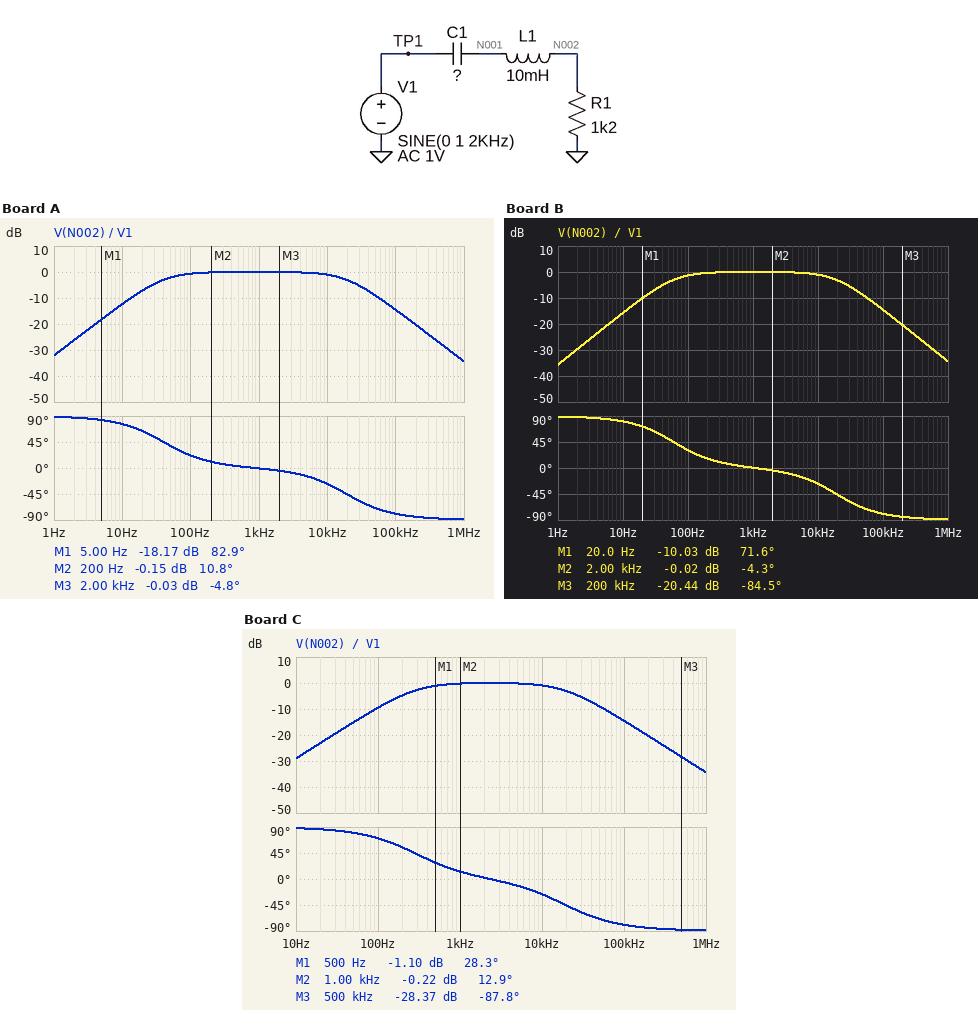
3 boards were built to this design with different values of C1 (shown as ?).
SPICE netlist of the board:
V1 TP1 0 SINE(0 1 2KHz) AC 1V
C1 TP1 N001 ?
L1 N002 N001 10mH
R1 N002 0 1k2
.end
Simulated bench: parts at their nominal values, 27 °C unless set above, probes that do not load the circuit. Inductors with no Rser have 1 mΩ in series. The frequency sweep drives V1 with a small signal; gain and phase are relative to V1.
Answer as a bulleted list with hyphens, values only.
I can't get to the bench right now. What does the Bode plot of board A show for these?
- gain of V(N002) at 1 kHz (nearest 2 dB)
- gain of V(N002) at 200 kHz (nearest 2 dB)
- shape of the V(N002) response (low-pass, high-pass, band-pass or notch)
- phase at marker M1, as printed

- 0 dB
- -20 dB
- band-pass
- 82.9 deg
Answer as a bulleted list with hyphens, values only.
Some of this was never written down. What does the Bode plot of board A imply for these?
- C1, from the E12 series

- 3.3 µF
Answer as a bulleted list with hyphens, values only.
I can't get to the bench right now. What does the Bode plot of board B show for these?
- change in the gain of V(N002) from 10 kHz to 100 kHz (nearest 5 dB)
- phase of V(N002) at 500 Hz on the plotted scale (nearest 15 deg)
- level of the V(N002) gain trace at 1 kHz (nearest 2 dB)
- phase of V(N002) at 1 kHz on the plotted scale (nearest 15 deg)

- -15 dB
- 0 deg
- 0 dB
- 0 deg
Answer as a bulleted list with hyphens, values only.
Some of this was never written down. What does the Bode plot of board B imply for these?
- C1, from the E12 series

- 2.2 µF
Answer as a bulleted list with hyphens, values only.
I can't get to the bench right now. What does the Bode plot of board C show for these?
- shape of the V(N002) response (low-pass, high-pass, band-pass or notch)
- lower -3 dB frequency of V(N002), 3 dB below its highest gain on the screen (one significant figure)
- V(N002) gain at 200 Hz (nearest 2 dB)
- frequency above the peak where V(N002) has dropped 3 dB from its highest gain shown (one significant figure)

- band-pass
- 300 Hz
- -4 dB
- 20 kHz
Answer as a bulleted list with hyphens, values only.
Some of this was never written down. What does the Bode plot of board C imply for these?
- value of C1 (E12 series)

- 470 nF
